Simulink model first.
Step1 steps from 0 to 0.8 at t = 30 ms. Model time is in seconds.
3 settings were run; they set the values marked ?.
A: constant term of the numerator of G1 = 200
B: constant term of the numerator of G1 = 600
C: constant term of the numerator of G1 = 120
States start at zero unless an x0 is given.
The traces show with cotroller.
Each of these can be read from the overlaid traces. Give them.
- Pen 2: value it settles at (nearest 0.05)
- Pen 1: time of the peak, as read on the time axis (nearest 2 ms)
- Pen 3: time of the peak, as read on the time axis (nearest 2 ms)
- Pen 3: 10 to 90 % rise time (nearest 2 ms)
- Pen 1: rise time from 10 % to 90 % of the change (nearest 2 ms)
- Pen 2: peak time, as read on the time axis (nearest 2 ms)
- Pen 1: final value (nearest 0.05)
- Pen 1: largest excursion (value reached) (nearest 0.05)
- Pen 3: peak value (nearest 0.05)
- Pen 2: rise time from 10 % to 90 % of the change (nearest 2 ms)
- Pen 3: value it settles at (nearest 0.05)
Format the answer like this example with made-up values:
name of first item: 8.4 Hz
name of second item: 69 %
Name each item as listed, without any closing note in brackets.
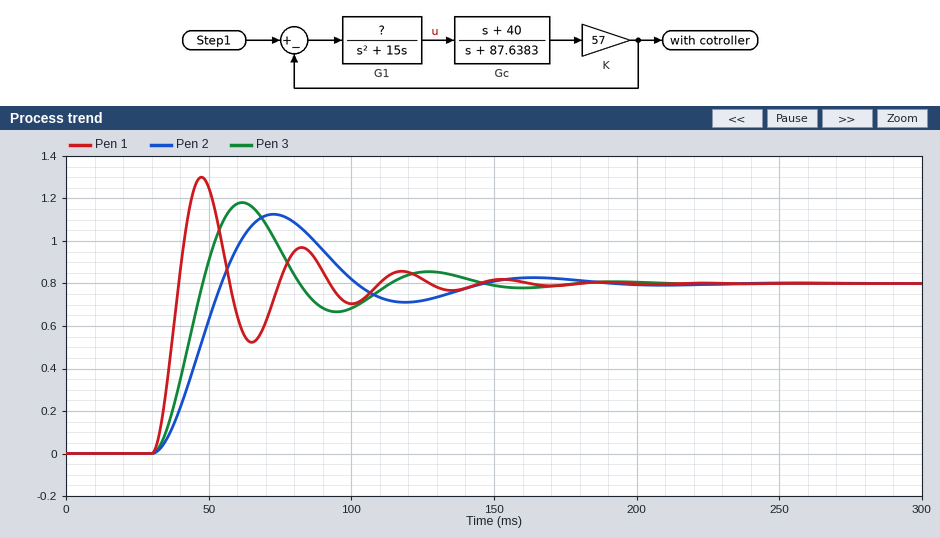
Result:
Pen 2: value it settles at: 0.80
Pen 1: time of the peak, as read on the time axis: 48 ms
Pen 3: time of the peak, as read on the time axis: 62 ms
Pen 3: 10 to 90 % rise time: 12 ms
Pen 1: rise time from 10 % to 90 % of the change: 6 ms
Pen 2: peak time, as read on the time axis: 72 ms
Pen 1: final value: 0.80
Pen 1: largest excursion (value reached): 1.30
Pen 3: peak value: 1.20
Pen 2: rise time from 10 % to 90 % of the change: 16 ms
Pen 3: value it settles at: 0.80
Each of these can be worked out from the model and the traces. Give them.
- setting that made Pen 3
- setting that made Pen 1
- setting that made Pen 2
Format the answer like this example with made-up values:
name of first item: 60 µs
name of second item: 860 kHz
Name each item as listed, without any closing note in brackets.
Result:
setting that made Pen 3: A
setting that made Pen 1: B
setting that made Pen 2: C
